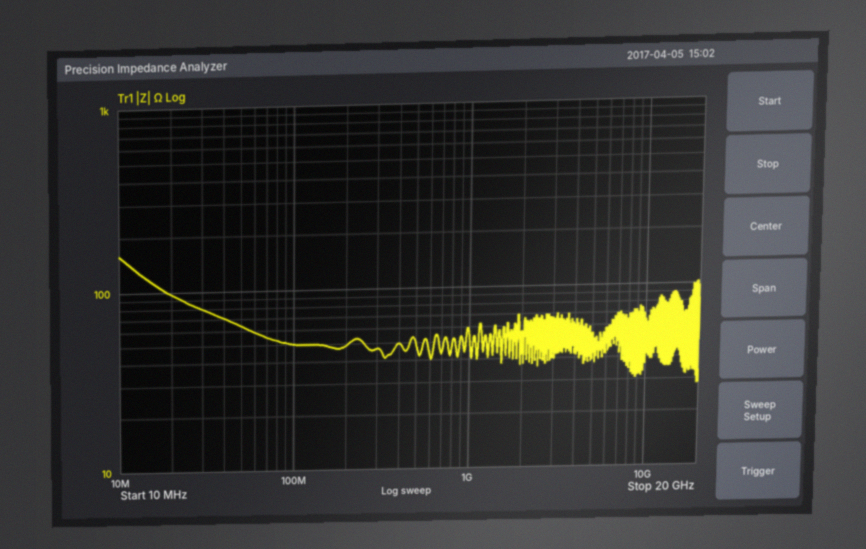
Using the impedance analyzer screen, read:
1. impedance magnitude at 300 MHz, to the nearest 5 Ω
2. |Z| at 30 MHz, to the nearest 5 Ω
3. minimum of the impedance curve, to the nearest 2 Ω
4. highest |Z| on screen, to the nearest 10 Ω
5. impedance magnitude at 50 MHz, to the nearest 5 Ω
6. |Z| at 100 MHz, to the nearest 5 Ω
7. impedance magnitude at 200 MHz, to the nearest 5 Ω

45 Ω
80 Ω
28 Ω
160 Ω
65 Ω
50 Ω
50 Ω
